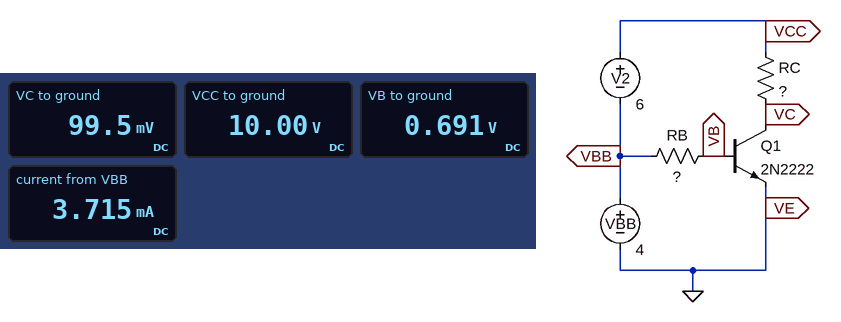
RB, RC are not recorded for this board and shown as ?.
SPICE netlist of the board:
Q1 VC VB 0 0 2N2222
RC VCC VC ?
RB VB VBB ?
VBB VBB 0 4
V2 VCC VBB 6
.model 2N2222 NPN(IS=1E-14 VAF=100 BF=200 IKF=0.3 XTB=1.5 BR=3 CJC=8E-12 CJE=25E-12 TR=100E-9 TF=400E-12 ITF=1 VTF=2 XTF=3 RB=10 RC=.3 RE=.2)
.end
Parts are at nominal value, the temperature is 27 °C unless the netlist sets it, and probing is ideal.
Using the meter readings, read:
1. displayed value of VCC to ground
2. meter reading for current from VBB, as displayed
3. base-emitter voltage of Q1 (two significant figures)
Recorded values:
10.00 V
3.715 mA
690 mV
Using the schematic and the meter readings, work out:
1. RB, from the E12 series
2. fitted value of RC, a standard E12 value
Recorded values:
68 kΩ
2.7 kΩ
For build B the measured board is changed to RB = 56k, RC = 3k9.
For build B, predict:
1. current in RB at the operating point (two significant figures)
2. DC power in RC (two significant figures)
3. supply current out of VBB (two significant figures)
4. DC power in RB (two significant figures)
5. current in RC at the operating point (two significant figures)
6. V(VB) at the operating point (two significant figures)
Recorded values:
59 µA
25 mW
2.6 mA
200 µW
2.5 mA
680 mV
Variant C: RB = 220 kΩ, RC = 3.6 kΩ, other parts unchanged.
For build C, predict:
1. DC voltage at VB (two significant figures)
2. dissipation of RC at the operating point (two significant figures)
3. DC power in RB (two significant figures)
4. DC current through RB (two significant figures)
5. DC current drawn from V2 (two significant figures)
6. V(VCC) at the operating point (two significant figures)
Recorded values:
680 mV
27 mW
50 µW
15 µA
2.7 mA
10 V
